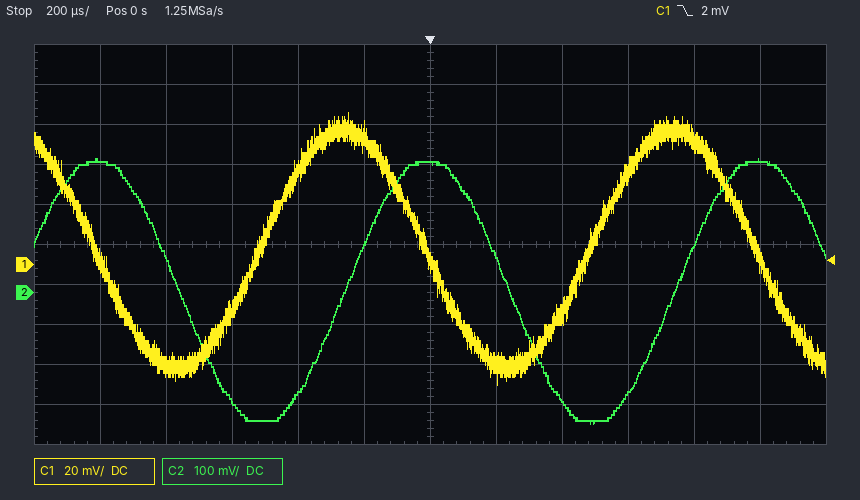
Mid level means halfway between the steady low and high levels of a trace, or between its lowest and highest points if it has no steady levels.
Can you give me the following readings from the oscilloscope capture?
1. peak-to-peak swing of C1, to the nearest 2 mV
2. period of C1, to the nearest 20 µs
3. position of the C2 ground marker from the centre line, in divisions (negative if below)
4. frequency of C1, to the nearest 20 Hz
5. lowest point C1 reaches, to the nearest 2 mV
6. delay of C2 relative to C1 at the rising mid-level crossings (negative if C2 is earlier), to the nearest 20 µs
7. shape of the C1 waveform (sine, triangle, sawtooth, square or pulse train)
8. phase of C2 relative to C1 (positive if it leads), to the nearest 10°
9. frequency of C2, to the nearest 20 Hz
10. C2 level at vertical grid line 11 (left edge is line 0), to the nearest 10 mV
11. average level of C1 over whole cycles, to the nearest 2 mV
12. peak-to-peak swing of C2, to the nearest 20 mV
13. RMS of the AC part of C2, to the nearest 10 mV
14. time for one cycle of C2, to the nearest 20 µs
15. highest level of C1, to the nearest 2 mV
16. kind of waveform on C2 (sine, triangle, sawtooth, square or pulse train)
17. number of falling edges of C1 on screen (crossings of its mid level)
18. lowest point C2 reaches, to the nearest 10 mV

136 mV
1.00 ms
-1.2 div
1.00 kHz
-60 mV
+260 µs
sine
-90°
1.00 kHz
330 mV
8 mV
660 mV
230 mV
1.00 ms
76 mV
sine
3
-330 mV
